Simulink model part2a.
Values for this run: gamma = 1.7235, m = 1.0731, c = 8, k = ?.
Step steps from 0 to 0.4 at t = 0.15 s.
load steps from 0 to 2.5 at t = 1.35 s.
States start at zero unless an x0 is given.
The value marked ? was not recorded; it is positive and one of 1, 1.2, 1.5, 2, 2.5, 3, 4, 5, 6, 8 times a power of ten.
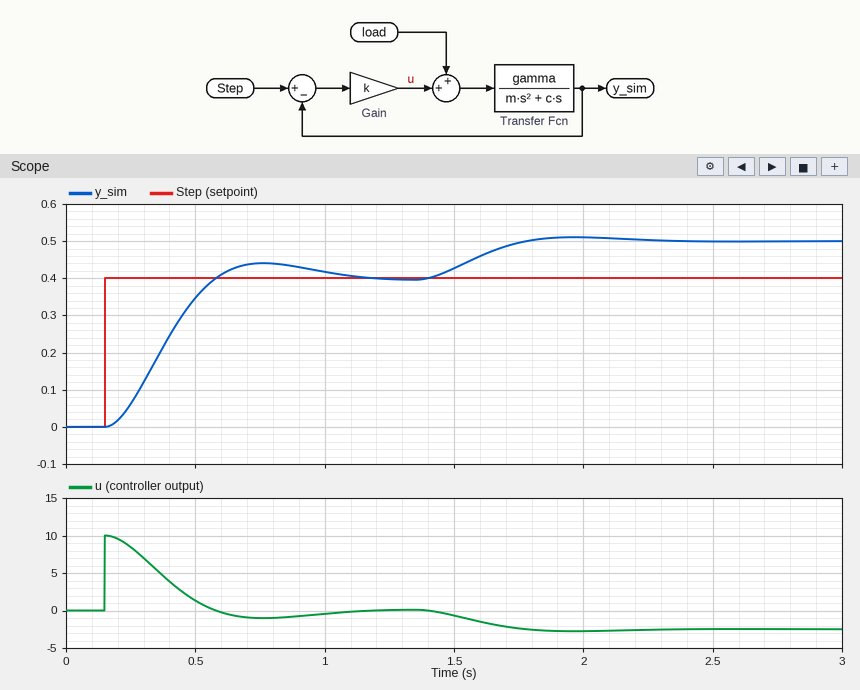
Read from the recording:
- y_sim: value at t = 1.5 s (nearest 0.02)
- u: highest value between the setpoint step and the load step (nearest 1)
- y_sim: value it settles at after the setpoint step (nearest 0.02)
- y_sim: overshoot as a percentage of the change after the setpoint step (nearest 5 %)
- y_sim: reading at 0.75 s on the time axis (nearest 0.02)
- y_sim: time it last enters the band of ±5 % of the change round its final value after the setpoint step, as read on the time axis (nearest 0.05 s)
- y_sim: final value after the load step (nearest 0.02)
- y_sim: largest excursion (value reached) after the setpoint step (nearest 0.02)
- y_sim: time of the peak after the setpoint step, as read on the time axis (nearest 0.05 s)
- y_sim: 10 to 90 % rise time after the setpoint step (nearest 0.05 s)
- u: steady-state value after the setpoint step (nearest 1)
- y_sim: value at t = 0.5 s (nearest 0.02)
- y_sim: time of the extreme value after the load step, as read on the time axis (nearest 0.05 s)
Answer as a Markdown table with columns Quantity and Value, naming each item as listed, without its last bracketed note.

| Quantity | Value |
|---|---|
| y_sim: value at t = 1.5 s | 0.42 |
| u: highest value between the setpoint step and the load step | 10 |
| y_sim: value it settles at after the setpoint step | 0.40 |
| y_sim: overshoot as a percentage of the change after the setpoint step | 10 % |
| y_sim: reading at 0.75 s on the time axis | 0.44 |
| y_sim: time it last enters the band of ±5 % of the change round its final value after the setpoint step, as read on the time axis | 1.00 s |
| y_sim: final value after the load step | 0.50 |
| y_sim: largest excursion (value reached) after the setpoint step | 0.44 |
| y_sim: time of the peak after the setpoint step, as read on the time axis | 0.75 s |
| y_sim: 10 to 90 % rise time after the setpoint step | 0.30 s |
| u: steady-state value after the setpoint step | 0 |
| y_sim: value at t = 0.5 s | 0.34 |
| y_sim: time of the extreme value after the load step, as read on the time axis | 1.95 s |
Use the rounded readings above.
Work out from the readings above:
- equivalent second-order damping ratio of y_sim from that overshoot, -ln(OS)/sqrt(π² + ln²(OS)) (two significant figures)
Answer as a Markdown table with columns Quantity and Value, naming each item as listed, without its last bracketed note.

| Quantity | Value |
|---|---|
| equivalent second-order damping ratio of y_sim from that overshoot, -ln(OS)/sqrt(π² + ln²(OS)) | 0.59 |
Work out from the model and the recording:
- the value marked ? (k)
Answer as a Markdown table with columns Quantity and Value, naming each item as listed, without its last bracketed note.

| Quantity | Value |
|---|---|
| the value marked ? | 25 |
